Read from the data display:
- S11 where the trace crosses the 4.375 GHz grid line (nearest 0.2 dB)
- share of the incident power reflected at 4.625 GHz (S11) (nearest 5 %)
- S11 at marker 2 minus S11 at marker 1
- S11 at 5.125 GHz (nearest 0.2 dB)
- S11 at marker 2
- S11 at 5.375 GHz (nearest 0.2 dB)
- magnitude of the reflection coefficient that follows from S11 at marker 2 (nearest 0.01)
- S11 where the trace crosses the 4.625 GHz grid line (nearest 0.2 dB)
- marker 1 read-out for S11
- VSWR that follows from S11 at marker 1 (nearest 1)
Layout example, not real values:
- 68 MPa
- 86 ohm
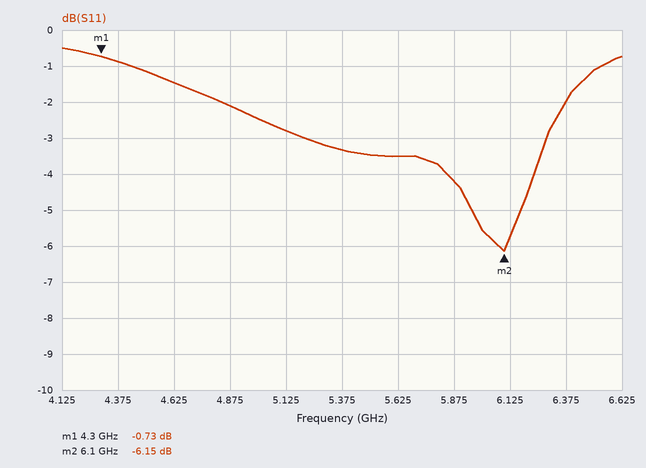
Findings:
- -0.8 dB
- 70 %
- -5.42 dB
- -2.8 dB
- -6.15 dB
- -3.4 dB
- 0.49
- -1.4 dB
- -0.73 dB
- 24
